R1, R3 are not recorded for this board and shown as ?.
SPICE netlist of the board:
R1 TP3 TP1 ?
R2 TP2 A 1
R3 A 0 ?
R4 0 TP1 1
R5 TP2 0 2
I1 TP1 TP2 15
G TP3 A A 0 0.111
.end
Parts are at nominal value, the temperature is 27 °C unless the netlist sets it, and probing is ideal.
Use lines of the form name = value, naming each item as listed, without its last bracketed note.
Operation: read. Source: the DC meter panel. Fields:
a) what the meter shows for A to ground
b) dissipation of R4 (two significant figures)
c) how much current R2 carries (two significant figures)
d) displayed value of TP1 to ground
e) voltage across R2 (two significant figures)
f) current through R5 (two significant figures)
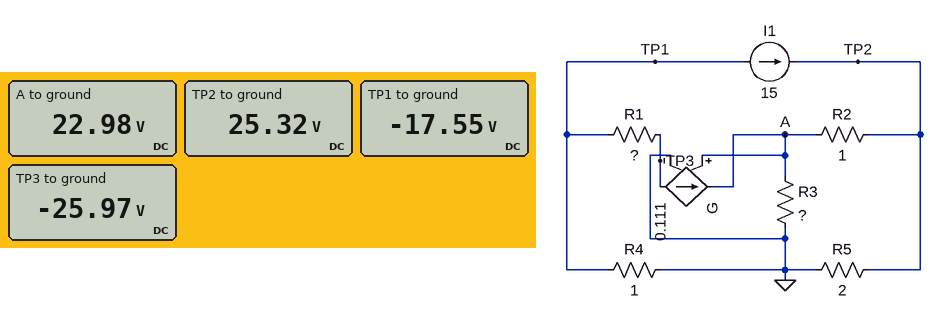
what the meter shows for A to ground = 22.98 V
dissipation of R4 = 310 W
how much current R2 carries = 2.3 A
displayed value of TP1 to ground = -17.55 V
voltage across R2 = 2.3 V
current through R5 = 13 A
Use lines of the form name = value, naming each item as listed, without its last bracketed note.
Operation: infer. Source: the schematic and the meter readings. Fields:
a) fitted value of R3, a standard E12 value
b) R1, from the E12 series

fitted value of R3, a standard E12 value = 4.7 Ω
R1, from the E12 series = 3.3 Ω
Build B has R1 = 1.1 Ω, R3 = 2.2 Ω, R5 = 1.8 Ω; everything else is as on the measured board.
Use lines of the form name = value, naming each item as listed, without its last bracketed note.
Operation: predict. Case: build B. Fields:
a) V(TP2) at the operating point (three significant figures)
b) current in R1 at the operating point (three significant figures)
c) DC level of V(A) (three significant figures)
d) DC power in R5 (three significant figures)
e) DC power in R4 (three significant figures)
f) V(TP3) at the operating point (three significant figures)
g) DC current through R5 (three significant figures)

V(TP2) at the operating point = 18.5 V
current in R1 at the operating point = 1.53 A
DC level of V(A) = 13.8 V
DC power in R5 = 190 W
DC power in R4 = 273 W
V(TP3) at the operating point = -18.2 V
DC current through R5 = 10.3 A
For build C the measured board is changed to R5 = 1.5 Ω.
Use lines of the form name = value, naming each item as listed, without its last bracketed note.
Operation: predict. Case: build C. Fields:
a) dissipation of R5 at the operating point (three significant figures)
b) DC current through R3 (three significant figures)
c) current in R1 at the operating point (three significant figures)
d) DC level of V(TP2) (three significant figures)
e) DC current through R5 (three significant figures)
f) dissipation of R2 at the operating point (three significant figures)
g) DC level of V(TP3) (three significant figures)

dissipation of R5 at the operating point = 260 W
DC current through R3 = 3.82 A
current in R1 at the operating point = 1.99 A
DC level of V(TP2) = 19.8 V
DC current through R5 = 13.2 A
dissipation of R2 at the operating point = 3.33 W
DC level of V(TP3) = -23.6 V
